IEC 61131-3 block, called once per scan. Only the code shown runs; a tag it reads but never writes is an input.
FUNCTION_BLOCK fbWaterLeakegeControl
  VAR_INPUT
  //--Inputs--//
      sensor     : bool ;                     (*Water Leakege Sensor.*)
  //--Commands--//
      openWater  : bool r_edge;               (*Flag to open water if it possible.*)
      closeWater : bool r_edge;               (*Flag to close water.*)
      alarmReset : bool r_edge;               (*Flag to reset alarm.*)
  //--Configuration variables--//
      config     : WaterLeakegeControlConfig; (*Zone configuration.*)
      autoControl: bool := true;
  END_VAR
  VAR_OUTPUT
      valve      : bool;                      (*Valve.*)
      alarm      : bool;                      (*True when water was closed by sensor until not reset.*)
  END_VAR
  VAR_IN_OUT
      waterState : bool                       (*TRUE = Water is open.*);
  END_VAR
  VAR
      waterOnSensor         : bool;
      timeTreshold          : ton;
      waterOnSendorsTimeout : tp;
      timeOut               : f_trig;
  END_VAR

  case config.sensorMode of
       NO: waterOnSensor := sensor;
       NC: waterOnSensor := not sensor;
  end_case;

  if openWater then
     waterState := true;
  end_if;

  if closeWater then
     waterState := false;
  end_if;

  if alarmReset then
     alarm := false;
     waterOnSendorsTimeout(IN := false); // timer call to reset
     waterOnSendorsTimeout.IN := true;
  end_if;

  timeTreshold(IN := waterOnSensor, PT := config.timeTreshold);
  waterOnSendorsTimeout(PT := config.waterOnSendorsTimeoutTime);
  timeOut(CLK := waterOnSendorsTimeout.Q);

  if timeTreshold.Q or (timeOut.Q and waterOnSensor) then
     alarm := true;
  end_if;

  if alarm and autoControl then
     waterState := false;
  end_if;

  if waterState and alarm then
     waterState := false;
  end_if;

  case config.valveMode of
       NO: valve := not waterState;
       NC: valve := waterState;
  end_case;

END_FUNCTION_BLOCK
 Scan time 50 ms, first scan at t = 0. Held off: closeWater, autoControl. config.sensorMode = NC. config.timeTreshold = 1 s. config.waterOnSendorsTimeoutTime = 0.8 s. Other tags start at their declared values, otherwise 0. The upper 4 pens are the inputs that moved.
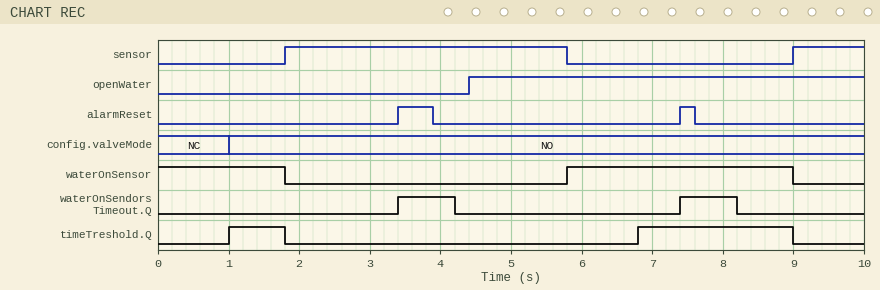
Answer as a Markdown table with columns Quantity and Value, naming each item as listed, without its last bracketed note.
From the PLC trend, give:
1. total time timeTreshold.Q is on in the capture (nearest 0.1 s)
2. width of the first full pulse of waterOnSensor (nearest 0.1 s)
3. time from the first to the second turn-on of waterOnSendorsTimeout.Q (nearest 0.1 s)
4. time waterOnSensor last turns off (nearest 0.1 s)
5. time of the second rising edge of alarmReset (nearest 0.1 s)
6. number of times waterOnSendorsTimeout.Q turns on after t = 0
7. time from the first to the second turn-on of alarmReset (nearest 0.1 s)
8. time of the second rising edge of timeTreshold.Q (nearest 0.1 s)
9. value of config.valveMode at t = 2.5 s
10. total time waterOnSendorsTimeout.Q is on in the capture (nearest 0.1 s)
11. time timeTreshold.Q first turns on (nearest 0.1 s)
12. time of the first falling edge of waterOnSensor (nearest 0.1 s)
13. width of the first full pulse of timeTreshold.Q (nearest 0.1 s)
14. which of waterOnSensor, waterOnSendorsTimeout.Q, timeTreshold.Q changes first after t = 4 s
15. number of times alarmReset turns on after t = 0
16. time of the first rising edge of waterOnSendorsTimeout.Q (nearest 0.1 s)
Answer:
| Quantity | Value |
|---|---|
| total time timeTreshold.Q is on in the capture | 3.0 s |
| width of the first full pulse of waterOnSensor | 3.2 s |
| time from the first to the second turn-on of waterOnSendorsTimeout.Q | 4.0 s |
| time waterOnSensor last turns off | 9.0 s |
| time of the second rising edge of alarmReset | 7.4 s |
| number of times waterOnSendorsTimeout.Q turns on after t = 0 | 2 |
| time from the first to the second turn-on of alarmReset | 4.0 s |
| time of the second rising edge of timeTreshold.Q | 6.8 s |
| value of config.valveMode at t = 2.5 s | NO |
| total time waterOnSendorsTimeout.Q is on in the capture | 1.6 s |
| time timeTreshold.Q first turns on | 1.0 s |
| time of the first falling edge of waterOnSensor | 1.8 s |
| width of the first full pulse of timeTreshold.Q | 0.8 s |
| which of waterOnSensor, waterOnSendorsTimeout.Q, timeTreshold.Q changes first after t = 4 s | waterOnSendorsTimeout.Q |
| number of times alarmReset turns on after t = 0 | 2 |
| time of the first rising edge of waterOnSendorsTimeout.Q | 3.4 s |
